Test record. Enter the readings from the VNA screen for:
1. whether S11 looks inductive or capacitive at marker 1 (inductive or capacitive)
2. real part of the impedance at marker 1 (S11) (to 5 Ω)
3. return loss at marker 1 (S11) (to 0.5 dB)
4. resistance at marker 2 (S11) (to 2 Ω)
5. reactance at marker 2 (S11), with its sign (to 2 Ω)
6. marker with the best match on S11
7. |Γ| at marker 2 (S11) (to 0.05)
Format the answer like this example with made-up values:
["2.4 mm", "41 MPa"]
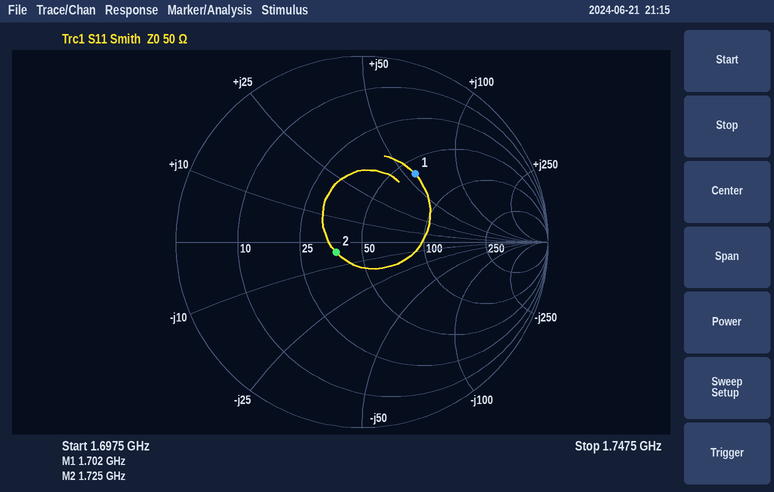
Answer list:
["inductive", "60 Ω", "6.5 dB", "38 Ω", "-4 Ω", "marker 2", "0.15"]
